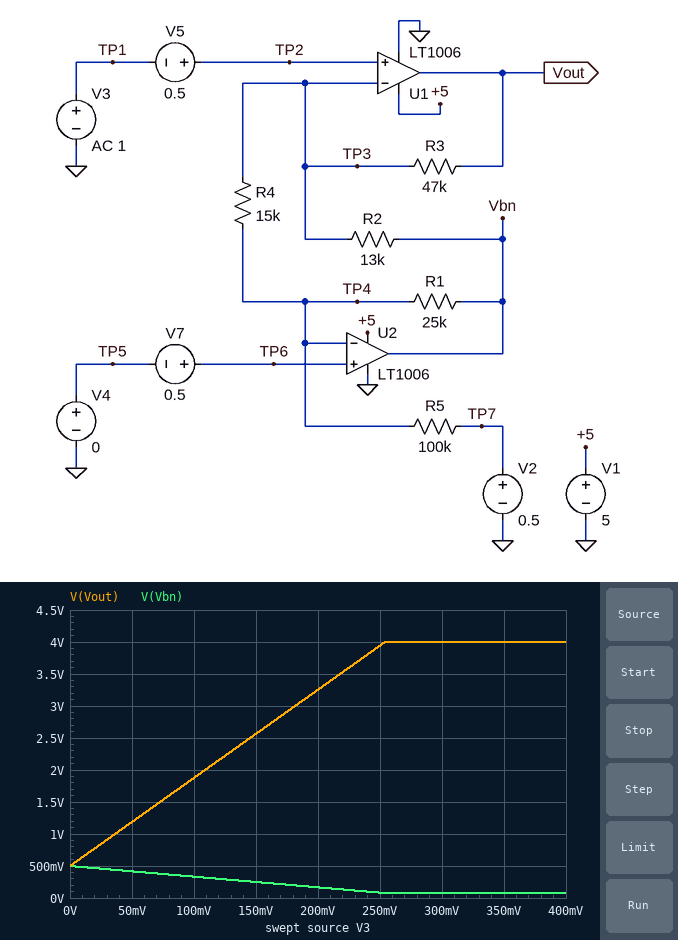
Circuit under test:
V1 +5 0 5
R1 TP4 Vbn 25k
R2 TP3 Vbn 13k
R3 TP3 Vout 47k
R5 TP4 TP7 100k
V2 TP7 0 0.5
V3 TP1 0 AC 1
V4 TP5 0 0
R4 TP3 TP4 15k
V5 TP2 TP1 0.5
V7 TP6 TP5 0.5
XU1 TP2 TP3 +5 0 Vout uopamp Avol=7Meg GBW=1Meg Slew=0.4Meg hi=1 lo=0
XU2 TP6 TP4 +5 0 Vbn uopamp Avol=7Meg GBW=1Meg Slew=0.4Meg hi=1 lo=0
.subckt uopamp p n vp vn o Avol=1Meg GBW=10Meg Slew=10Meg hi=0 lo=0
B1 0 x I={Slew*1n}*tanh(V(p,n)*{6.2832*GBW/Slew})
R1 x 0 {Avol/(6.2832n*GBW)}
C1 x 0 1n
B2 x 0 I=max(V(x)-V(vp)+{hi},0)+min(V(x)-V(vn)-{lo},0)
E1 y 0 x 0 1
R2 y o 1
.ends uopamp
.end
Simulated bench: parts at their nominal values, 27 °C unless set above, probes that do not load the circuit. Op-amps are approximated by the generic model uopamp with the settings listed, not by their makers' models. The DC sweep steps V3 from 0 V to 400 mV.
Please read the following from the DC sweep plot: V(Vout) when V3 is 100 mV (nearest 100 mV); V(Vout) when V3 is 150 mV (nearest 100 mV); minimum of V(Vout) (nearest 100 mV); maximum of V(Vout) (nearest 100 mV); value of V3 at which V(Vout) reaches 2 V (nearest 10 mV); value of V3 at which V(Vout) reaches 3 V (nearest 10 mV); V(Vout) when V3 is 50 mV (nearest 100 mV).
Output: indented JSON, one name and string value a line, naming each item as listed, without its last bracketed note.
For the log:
{
  "V(Vout) when V3 is 100 mV": "1.9 V",
  "V(Vout) when V3 is 150 mV": "2.6 V",
  "minimum of V(Vout)": "500 mV",
  "maximum of V(Vout)": "4.0 V",
  "value of V3 at which V(Vout) reaches 2 V": "110 mV",
  "value of V3 at which V(Vout) reaches 3 V": "180 mV",
  "V(Vout) when V3 is 50 mV": "1.2 V"
}
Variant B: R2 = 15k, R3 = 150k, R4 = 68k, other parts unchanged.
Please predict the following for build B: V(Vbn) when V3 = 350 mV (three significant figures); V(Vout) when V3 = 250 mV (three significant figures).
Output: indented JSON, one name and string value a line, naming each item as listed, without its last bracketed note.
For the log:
{
  "V(Vbn) when V3 = 350 mV": "424 mV",
  "V(Vout) when V3 = 250 mV": "4.00 V"
}
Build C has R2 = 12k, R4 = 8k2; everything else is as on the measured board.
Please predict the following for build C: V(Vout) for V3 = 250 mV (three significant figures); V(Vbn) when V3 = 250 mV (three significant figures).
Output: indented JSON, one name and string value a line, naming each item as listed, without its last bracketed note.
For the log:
{
  "V(Vout) for V3 = 250 mV": "4.00 V",
  "V(Vbn) when V3 = 250 mV": "27.6 mV"
}
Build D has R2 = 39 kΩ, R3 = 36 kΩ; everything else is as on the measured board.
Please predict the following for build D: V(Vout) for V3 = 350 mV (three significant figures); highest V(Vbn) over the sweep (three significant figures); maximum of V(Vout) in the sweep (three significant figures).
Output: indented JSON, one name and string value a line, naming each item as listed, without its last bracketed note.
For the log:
{
  "V(Vout) for V3 = 350 mV": "2.41 V",
  "highest V(Vbn) over the sweep": "500 mV",
  "maximum of V(Vout) in the sweep": "2.55 V"
}
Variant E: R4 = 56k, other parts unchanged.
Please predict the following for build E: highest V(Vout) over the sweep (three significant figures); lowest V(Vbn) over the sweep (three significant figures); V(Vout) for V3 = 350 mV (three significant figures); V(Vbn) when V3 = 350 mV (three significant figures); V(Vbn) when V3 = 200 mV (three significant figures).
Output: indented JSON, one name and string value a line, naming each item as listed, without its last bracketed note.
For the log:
{
  "highest V(Vout) over the sweep": "3.33 V",
  "lowest V(Vbn) over the sweep": "321 mV",
  "V(Vout) for V3 = 350 mV": "2.97 V",
  "V(Vbn) when V3 = 350 mV": "344 mV",
  "V(Vbn) when V3 = 200 mV": "411 mV"
}
